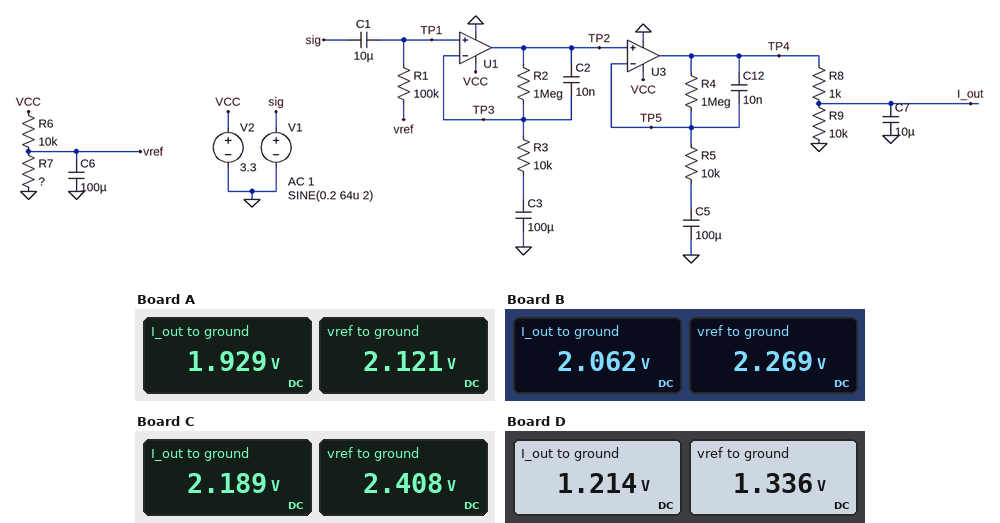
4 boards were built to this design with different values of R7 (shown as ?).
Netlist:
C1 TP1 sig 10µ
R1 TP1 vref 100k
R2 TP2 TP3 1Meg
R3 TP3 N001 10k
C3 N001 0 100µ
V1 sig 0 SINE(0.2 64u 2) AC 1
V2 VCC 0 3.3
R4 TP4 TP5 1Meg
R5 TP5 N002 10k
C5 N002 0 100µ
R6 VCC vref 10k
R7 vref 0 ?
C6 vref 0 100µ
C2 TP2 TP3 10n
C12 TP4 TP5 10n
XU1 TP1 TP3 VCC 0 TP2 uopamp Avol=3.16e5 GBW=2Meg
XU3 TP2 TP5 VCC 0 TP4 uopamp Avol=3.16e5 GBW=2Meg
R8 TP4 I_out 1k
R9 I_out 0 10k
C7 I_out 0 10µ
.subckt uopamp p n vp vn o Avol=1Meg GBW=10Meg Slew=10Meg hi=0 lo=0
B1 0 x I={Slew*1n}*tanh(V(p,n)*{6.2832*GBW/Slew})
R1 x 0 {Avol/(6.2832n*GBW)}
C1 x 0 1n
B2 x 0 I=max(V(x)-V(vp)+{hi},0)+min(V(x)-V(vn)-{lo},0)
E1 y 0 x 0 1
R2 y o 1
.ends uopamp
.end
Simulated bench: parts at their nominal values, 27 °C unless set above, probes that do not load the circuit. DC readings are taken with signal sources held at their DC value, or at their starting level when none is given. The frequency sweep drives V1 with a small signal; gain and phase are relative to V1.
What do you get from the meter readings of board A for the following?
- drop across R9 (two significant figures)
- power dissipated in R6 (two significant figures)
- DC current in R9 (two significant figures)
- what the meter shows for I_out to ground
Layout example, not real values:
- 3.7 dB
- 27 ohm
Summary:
- 1.9 V
- 140 µW
- 190 µA
- 1.929 V
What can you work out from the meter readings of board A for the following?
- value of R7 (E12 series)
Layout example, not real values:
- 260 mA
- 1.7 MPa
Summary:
- 18 kΩ
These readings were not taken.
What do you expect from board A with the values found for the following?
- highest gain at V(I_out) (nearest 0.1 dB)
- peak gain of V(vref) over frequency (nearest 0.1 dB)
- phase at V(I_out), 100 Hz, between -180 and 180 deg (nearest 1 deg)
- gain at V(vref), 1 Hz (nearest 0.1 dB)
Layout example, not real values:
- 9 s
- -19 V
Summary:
- 79.1 dB
- -28.5 dB
- 125 deg
- -36.4 dB
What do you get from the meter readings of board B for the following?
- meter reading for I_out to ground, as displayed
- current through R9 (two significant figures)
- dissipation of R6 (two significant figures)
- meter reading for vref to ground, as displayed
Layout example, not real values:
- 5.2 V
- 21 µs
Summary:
- 2.062 V
- 210 µA
- 110 µW
- 2.269 V
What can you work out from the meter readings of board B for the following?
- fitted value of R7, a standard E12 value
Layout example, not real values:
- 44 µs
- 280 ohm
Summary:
- 22 kΩ
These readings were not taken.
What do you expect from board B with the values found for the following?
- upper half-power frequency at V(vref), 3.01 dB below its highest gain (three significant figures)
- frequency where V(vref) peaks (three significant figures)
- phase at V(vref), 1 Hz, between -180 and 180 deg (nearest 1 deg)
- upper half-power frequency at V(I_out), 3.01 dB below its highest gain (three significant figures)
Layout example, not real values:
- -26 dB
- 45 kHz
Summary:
- 483 mHz
- 192 mHz
- -67 deg
- 8.75 Hz
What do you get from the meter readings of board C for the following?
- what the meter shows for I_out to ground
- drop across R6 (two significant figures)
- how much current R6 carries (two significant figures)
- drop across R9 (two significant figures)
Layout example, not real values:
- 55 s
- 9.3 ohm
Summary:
- 2.189 V
- 890 mV
- 89 µA
- 2.2 V
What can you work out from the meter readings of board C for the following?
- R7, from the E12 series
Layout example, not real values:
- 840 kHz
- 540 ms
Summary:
- 27 kΩ
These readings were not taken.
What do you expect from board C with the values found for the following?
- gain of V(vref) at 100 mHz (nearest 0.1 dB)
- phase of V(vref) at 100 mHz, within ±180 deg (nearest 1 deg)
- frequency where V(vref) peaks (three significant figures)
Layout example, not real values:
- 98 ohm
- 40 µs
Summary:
- -29.3 dB
- 32 deg
- 186 mHz
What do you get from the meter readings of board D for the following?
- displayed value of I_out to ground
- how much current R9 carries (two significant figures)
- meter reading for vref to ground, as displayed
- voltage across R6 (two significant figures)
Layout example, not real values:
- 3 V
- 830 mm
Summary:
- 1.214 V
- 120 µA
- 1.336 V
- 2.0 V
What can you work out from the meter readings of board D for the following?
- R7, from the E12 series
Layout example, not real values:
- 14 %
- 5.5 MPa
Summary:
- 6.8 kΩ
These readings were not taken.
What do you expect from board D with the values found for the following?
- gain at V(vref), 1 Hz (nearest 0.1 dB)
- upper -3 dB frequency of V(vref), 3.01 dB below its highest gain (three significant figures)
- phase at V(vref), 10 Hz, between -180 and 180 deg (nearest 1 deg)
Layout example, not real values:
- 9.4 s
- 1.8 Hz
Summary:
- -36.8 dB
- 663 mHz
- -87 deg
